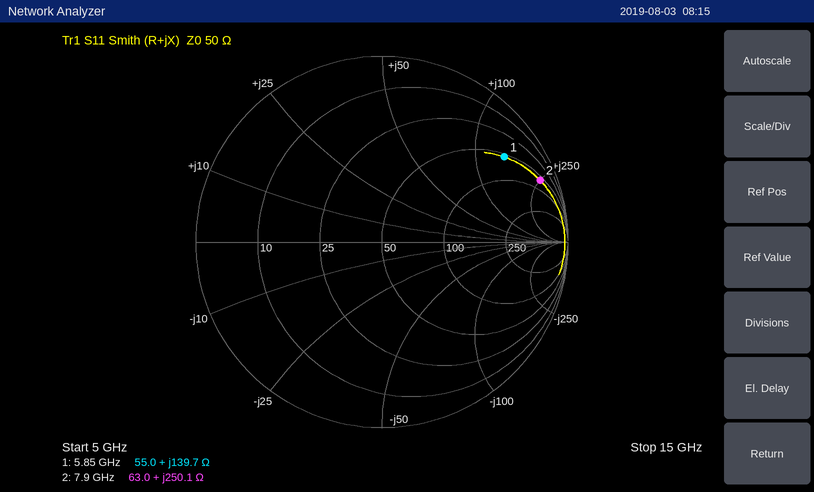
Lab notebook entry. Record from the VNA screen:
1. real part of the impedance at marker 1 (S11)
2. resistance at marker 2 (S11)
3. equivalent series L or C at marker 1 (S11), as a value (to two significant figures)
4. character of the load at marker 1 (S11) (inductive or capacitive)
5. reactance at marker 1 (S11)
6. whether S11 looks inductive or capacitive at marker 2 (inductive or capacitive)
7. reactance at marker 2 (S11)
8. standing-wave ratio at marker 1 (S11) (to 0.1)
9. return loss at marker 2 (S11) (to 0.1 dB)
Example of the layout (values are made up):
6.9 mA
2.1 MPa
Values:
55.0 Ω
63.0 Ω
3.8 nH
inductive
+139.7 Ω
inductive
+250.1 Ω
9.0
0.8 dB
